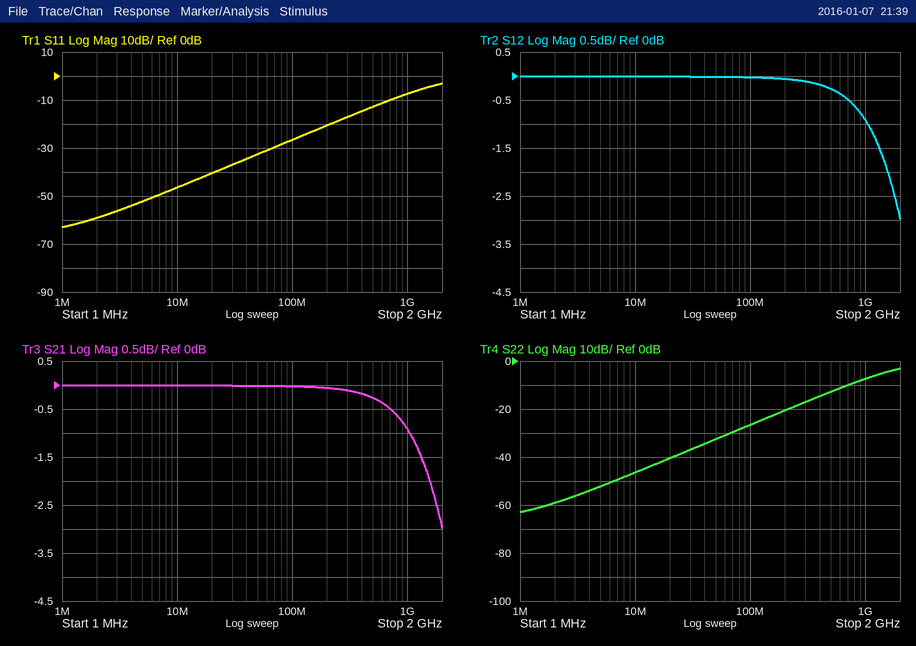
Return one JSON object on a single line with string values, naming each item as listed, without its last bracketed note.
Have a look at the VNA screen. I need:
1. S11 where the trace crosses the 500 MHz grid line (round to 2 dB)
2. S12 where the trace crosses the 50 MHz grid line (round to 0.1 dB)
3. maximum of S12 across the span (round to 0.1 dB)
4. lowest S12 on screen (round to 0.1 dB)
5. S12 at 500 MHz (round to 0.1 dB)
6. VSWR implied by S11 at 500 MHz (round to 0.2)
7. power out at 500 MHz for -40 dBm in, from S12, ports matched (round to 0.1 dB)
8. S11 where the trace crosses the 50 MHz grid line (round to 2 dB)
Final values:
{"S11 where the trace crosses the 500 MHz grid line": "-12 dB", "S12 where the trace crosses the 50 MHz grid line": "0.0 dB", "maximum of S12 across the span": "0.0 dB", "lowest S12 on screen": "-3.0 dB", "S12 at 500 MHz": "-0.3 dB", "VSWR implied by S11 at 500 MHz": "1.6", "power out at 500 MHz for -40 dBm in, from S12, ports matched": "-40.3 dBm", "S11 where the trace crosses the 50 MHz grid line": "-32 dB"}
